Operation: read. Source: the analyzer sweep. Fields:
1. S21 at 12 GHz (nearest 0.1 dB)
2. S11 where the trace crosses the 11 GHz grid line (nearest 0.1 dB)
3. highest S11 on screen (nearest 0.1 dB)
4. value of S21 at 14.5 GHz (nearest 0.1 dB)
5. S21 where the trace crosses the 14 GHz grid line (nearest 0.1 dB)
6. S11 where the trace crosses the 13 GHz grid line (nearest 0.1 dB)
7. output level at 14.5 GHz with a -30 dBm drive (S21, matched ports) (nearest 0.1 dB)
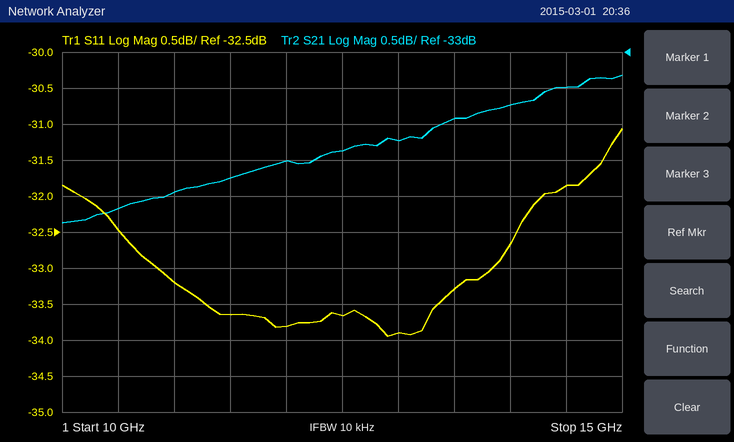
-34.5 dB
-33.2 dB
-31.1 dB
-33.5 dB
-33.7 dB
-33.9 dB
-63.5 dBm
